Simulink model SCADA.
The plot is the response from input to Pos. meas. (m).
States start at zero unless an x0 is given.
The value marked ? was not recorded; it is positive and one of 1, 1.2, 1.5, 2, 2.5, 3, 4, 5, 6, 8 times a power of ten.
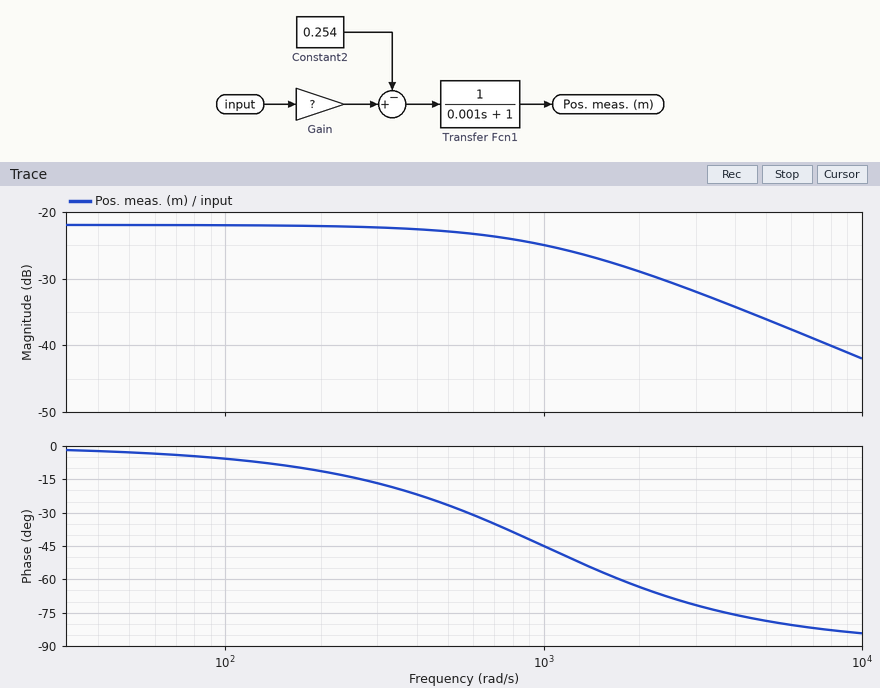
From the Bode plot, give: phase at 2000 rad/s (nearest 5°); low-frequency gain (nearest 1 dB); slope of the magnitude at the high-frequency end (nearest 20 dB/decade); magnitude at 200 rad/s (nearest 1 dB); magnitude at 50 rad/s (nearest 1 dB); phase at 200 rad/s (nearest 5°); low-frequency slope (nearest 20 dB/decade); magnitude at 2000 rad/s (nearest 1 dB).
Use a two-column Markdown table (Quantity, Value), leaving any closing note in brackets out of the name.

| Quantity | Value |
|---|---|
| phase at 2000 rad/s | -65° |
| low-frequency gain | -22 dB |
| slope of the magnitude at the high-frequency end | -20 dB/decade |
| magnitude at 200 rad/s | -22 dB |
| magnitude at 50 rad/s | -22 dB |
| phase at 200 rad/s | -10° |
| low-frequency slope | 0 dB/decade |
| magnitude at 2000 rad/s | -29 dB |
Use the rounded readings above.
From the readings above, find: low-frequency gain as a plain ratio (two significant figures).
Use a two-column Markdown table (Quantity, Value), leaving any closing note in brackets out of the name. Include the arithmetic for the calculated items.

| Quantity | Value |
|---|---|
| low-frequency gain as a plain ratio | 10^(-22 / 20) = 0.079 |
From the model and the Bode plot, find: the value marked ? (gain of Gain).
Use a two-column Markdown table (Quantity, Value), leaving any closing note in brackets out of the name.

| Quantity | Value |
|---|---|
| the value marked ? | 0.08 |
